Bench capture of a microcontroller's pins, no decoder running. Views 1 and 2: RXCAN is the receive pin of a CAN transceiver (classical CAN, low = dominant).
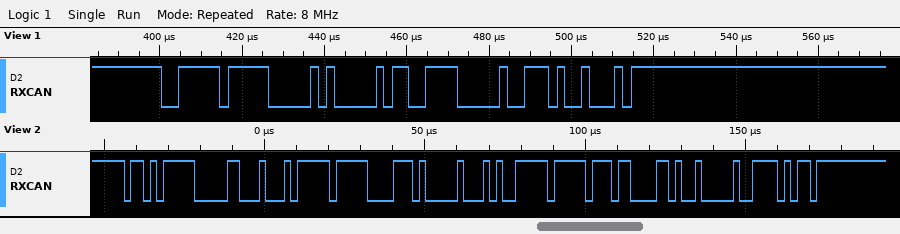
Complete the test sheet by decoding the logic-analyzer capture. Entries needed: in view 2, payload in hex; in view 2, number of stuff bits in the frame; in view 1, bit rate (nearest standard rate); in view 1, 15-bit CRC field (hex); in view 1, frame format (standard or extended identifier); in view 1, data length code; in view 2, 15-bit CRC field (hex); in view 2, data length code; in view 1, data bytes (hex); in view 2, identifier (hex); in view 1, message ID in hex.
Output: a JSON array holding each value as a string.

["8B FF 1D 00 A7 FF D8 69", "8", "500 kbit/s", "0x0748", "standard", "2", "0x00F5", "8", "06 78", "0x6BE", "0x3FF"]
